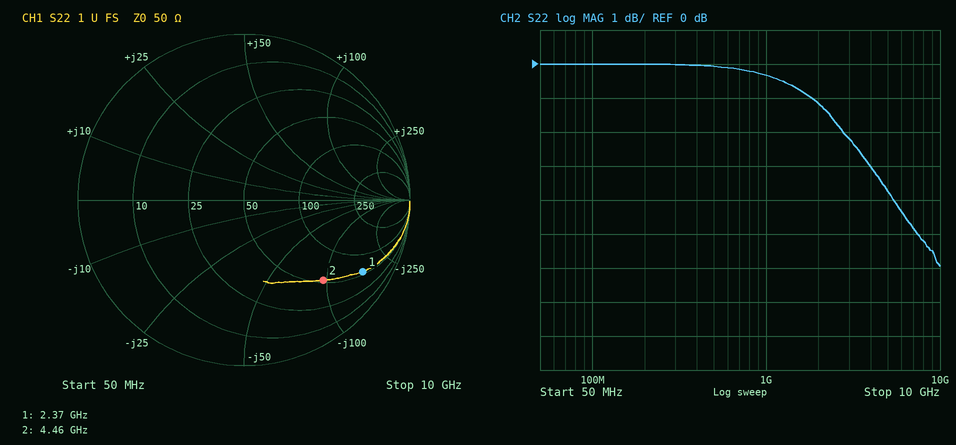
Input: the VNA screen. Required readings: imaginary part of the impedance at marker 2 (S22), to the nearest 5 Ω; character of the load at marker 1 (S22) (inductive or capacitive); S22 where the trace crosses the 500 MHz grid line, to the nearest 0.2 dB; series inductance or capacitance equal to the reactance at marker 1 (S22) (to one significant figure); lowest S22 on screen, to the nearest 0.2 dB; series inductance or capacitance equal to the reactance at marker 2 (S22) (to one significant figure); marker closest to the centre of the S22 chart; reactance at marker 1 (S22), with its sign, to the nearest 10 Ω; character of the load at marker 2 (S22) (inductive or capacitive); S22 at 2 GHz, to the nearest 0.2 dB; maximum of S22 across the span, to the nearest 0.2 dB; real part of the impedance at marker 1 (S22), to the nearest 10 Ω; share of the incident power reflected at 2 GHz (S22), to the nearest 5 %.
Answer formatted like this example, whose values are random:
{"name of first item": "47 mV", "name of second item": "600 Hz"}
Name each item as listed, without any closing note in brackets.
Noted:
{"imaginary part of the impedance at marker 2 (S22), to the nearest 5 Ω": "-95 Ω", "character of the load at marker 1 (S22)": "capacitive", "S22 where the trace crosses the 500 MHz grid line, to the nearest 0.2 dB": "0.0 dB", "series inductance or capacitance equal to the reactance at marker 1 (S22)": "400 fF", "lowest S22 on screen, to the nearest 0.2 dB": "-6.0 dB", "series inductance or capacitance equal to the reactance at marker 2 (S22)": "400 fF", "marker closest to the centre of the S22 chart": "marker 2", "reactance at marker 1 (S22), with its sign, to the nearest 10 Ω": "-160 Ω", "character of the load at marker 2 (S22)": "capacitive", "S22 at 2 GHz, to the nearest 0.2 dB": "-1.2 dB", "maximum of S22 across the span, to the nearest 0.2 dB": "0.0 dB", "real part of the impedance at marker 1 (S22), to the nearest 10 Ω": "60 Ω", "share of the incident power reflected at 2 GHz (S22), to the nearest 5 %": "75 %"}
